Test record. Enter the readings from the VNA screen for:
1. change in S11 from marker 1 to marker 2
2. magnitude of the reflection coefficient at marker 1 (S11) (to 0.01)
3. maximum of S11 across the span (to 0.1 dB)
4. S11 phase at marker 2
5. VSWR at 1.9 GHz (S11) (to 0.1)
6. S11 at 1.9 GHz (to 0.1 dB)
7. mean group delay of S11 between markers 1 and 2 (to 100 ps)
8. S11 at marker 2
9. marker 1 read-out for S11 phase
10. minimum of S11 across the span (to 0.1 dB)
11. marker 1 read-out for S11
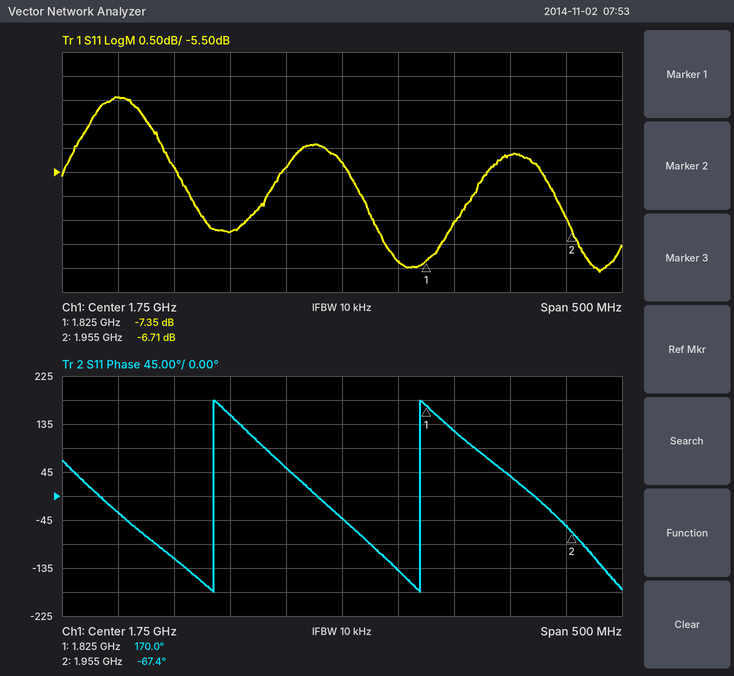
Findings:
0.64 dB
0.43
-3.9 dB
-67.4°
3.5
-5.1 dB
5.1 ns
-6.71 dB
170.0°
-7.6 dB
-7.35 dB
